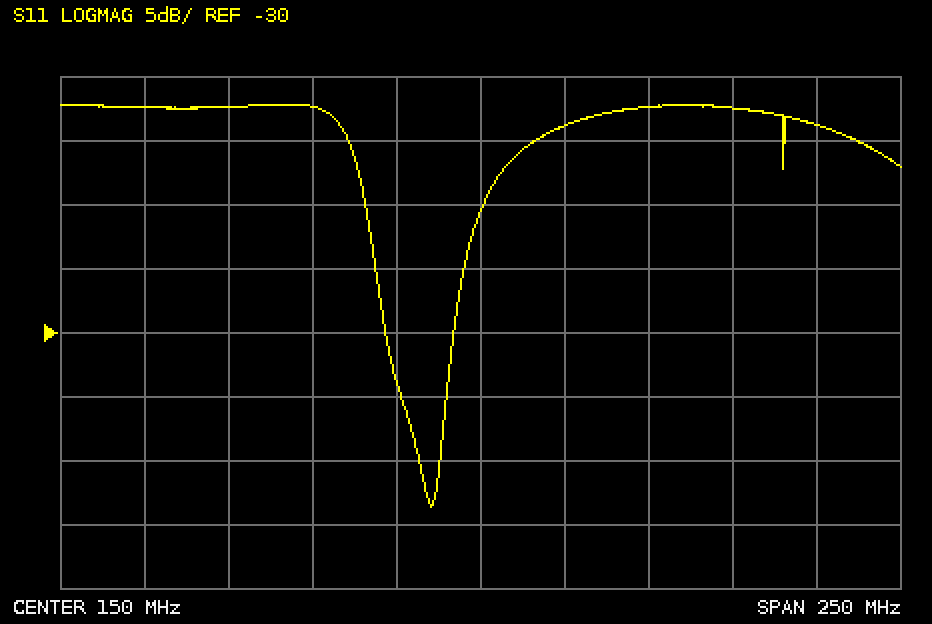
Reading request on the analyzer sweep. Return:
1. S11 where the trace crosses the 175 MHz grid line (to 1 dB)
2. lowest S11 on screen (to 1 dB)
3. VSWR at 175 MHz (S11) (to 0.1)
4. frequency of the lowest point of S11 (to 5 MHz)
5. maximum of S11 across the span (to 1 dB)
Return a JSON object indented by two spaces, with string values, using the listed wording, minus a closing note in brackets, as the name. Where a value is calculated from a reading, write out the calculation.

{
  "S11 where the trace crosses the 175 MHz grid line": "-14 dB",
  "lowest S11 on screen": "-44 dB",
  "VSWR at 175 MHz (S11)": "|Γ| = 10^(-14/20) = 0.1995; VSWR = (1 + 0.1995)/(1 − 0.1995) ≈ 1.5",
  "frequency of the lowest point of S11": "135 MHz",
  "maximum of S11 across the span": "-12 dB"
}
